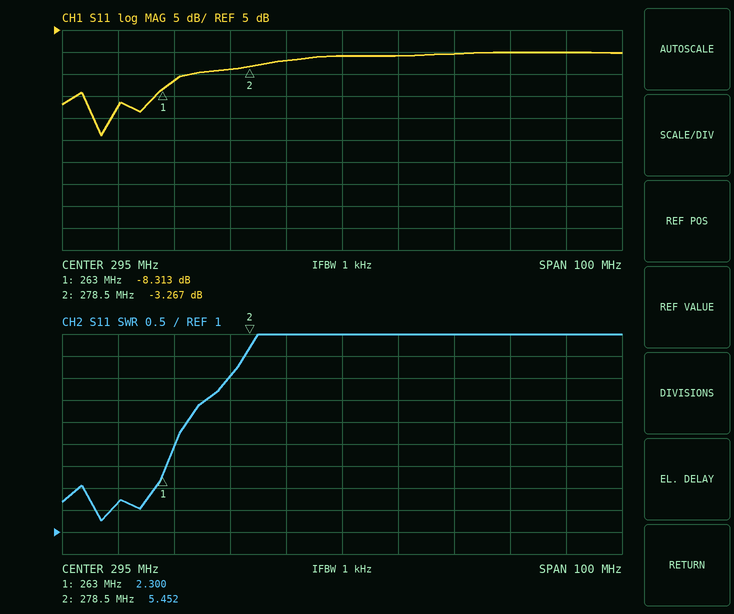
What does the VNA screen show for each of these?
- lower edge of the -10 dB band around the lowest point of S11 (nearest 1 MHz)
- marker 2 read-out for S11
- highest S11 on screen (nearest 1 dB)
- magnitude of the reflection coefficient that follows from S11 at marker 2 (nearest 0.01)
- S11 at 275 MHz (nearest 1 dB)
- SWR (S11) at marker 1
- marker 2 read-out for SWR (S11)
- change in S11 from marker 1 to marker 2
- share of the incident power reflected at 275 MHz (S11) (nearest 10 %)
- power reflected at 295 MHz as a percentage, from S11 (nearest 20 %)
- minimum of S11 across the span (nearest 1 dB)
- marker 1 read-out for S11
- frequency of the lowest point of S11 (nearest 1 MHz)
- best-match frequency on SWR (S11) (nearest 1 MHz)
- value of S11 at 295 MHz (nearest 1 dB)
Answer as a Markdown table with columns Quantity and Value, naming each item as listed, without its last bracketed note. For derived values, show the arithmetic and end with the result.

| Quantity | Value |
|---|---|
| lower edge of the -10 dB band around the lowest point of S11 | 249 MHz |
| marker 2 read-out for S11 | -3.267 dB |
| highest S11 on screen | 0 dB |
| magnitude of the reflection coefficient that follows from S11 at marker 2 | 10^(-3.267/20) ≈ 0.69 |
| S11 at 275 MHz | -4 dB |
| SWR (S11) at marker 1 | 2.300 |
| marker 2 read-out for SWR | 5.452 |
| change in S11 from marker 1 to marker 2 | -3.267 − (-8.313) = 5.046 dB |
| share of the incident power reflected at 275 MHz (S11) | 10^(-4/10) ≈ 40 % |
| power reflected at 295 MHz as a percentage, from S11 | 10^(-1/10) ≈ 79.4 %, so 80 % to the nearest 20 % |
| minimum of S11 across the span | -19 dB |
| marker 1 read-out for S11 | -8.313 dB |
| frequency of the lowest point of S11 | 252 MHz |
| best-match frequency on SWR (S11) | 252 MHz |
| value of S11 at 295 MHz | -1 dB |
